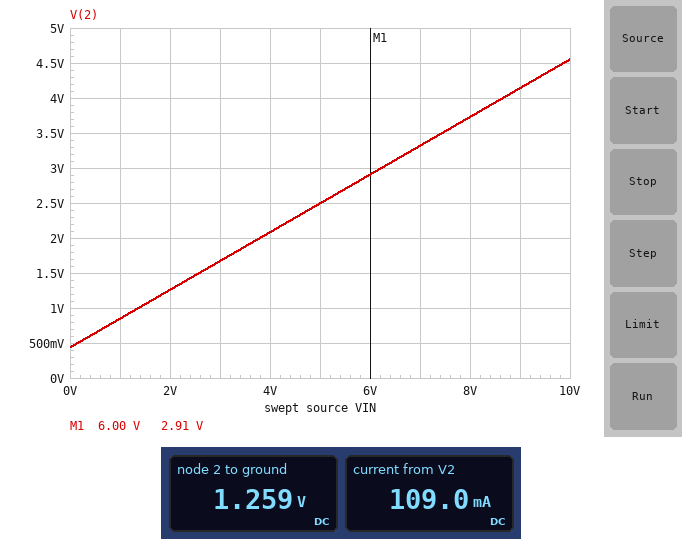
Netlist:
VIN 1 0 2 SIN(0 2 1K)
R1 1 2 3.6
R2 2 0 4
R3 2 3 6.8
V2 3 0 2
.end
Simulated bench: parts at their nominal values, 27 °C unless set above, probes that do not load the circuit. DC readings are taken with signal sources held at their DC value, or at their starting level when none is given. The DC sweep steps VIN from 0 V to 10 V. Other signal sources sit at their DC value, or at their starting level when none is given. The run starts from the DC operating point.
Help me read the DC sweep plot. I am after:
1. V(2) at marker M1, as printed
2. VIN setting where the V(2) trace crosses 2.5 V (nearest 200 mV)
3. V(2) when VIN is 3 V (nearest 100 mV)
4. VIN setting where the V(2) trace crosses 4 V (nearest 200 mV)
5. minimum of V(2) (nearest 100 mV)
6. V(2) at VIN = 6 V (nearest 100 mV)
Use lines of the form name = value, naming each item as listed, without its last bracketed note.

V(2) at marker M1, as printed = 2.91 V
VIN setting where the V(2) trace crosses 2.5 V = 5.0 V
V(2) when VIN is 3 V = 1.7 V
VIN setting where the V(2) trace crosses 4 V = 8.6 V
minimum of V(2) = 400 mV
V(2) at VIN = 6 V = 2.9 V
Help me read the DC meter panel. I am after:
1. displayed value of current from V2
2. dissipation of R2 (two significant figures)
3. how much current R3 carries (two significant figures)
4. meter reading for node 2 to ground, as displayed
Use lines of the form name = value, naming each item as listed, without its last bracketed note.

displayed value of current from V2 = 109.0 mA
dissipation of R2 = 400 mW
how much current R3 carries = 110 mA
meter reading for node 2 to ground, as displayed = 1.259 V
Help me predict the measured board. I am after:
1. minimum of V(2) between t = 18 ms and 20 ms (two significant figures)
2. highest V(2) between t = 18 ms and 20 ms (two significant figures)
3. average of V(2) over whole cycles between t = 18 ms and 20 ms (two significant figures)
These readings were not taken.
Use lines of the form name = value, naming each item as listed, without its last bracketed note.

minimum of V(2) between t = 18 ms and 20 ms = -390 mV
highest V(2) between t = 18 ms and 20 ms = 1.3 V
average of V(2) over whole cycles between t = 18 ms and 20 ms = 440 mV
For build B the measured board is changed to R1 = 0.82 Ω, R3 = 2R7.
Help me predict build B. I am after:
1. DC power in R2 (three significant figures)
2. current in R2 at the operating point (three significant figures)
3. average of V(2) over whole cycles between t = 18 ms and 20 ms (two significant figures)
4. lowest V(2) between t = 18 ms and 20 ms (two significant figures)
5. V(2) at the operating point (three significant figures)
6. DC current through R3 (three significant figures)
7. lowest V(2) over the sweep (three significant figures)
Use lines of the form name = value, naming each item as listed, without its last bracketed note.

DC power in R2 = 747 mW
current in R2 at the operating point = 432 mA
average of V(2) over whole cycles between t = 18 ms and 20 ms = 400 mV
lowest V(2) between t = 18 ms and 20 ms = -920 mV
V(2) at the operating point = 1.73 V
DC current through R3 = 101 mA
lowest V(2) over the sweep = 403 mV
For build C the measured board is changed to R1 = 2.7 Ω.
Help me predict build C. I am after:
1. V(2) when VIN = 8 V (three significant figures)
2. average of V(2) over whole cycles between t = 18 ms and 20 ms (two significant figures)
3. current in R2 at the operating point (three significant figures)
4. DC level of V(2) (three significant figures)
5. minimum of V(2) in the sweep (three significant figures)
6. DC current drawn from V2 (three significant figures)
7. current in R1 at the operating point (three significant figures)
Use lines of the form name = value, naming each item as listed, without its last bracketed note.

V(2) when VIN = 8 V = 4.24 V
average of V(2) over whole cycles between t = 18 ms and 20 ms = 380 mV
current in R2 at the operating point = 337 mA
DC level of V(2) = 1.35 V
minimum of V(2) in the sweep = 383 mV
DC current drawn from V2 = 95.8 mA
current in R1 at the operating point = 241 mA
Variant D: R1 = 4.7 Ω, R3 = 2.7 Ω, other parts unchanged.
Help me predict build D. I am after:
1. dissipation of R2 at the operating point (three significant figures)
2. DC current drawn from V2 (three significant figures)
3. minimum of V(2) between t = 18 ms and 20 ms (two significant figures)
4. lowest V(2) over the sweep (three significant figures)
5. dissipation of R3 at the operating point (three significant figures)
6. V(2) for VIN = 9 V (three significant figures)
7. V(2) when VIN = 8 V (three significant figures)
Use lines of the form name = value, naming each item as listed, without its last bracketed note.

dissipation of R2 at the operating point = 490 mW
DC current drawn from V2 = 222 mA
minimum of V(2) between t = 18 ms and 20 ms = 380 mV
lowest V(2) over the sweep = 889 mV
dissipation of R3 at the operating point = 133 mW
V(2) for VIN = 9 V = 3.19 V
V(2) when VIN = 8 V = 2.93 V
